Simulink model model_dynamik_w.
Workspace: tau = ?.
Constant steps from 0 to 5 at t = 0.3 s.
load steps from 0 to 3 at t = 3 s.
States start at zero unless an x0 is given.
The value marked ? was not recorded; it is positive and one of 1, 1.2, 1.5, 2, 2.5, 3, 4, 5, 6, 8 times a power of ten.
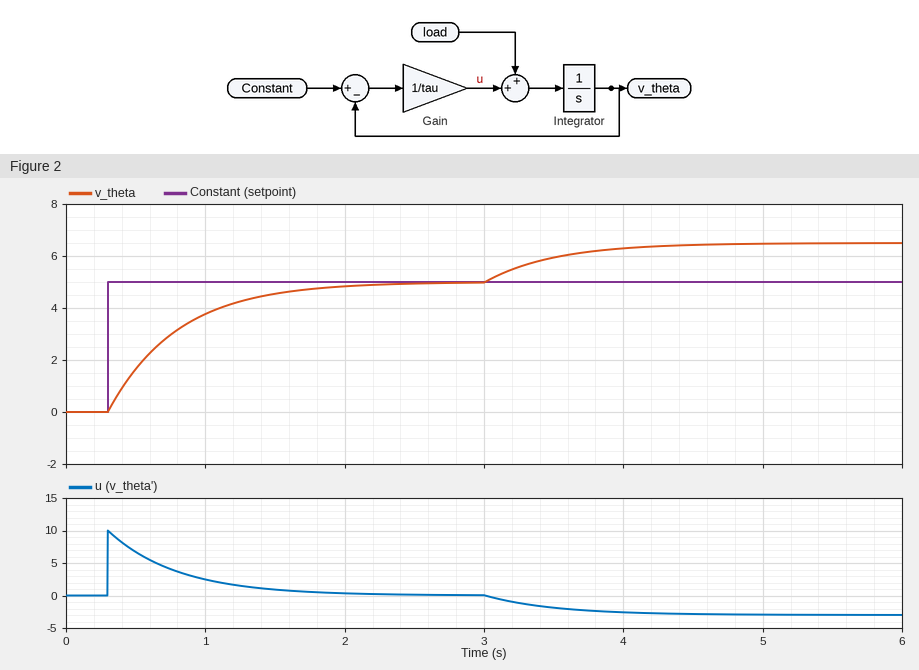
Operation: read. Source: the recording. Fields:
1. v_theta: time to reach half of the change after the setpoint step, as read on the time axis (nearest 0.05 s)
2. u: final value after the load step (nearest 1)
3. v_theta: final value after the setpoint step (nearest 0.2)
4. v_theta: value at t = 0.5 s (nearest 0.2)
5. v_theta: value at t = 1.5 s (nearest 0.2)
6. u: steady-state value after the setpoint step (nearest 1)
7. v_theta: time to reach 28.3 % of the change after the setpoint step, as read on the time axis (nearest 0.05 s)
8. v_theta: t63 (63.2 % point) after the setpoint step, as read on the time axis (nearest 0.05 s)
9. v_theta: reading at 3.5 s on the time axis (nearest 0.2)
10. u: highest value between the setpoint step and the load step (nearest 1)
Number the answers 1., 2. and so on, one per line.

1. 0.65 s
2. -3
3. 5.0
4. 1.6
5. 4.6
6. 0
7. 0.45 s
8. 0.80 s
9. 6.0
10. 10
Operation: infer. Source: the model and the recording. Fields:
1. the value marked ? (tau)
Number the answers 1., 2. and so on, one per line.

1. 0.5
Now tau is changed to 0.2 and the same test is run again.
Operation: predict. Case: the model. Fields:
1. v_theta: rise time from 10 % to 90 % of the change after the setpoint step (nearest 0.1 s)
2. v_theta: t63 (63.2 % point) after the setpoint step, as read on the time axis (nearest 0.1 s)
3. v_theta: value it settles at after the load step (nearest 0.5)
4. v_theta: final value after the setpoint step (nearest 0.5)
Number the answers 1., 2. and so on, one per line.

1. 0.4 s
2. 0.5 s
3. 5.5
4. 5.0
